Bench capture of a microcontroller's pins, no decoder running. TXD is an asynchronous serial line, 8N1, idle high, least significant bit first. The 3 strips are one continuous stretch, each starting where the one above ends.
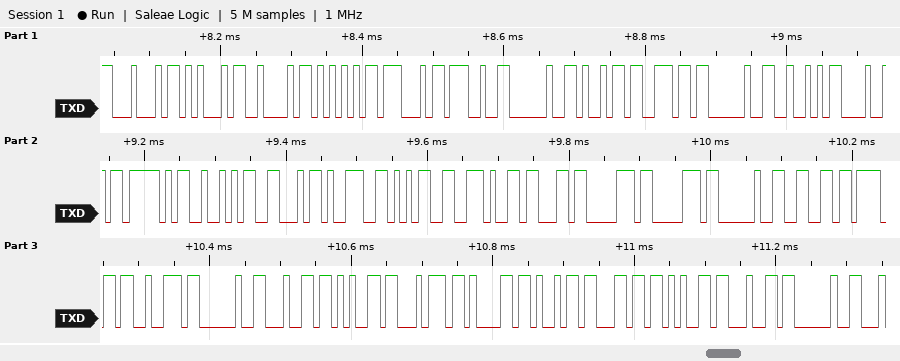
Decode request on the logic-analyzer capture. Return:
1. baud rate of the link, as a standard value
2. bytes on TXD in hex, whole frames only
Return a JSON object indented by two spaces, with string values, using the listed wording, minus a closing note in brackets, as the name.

{
  "baud rate of the link, as a standard value": "115200 baud",
  "bytes on TXD in hex, whole frames only": "44 45 42 55 47 27 20 69 6E 20 52 48 5F 52 46 39 35 2E 63 70 70 20 66 6F 72 20 64 65 74 61 69 6C 65 64 20"
}
